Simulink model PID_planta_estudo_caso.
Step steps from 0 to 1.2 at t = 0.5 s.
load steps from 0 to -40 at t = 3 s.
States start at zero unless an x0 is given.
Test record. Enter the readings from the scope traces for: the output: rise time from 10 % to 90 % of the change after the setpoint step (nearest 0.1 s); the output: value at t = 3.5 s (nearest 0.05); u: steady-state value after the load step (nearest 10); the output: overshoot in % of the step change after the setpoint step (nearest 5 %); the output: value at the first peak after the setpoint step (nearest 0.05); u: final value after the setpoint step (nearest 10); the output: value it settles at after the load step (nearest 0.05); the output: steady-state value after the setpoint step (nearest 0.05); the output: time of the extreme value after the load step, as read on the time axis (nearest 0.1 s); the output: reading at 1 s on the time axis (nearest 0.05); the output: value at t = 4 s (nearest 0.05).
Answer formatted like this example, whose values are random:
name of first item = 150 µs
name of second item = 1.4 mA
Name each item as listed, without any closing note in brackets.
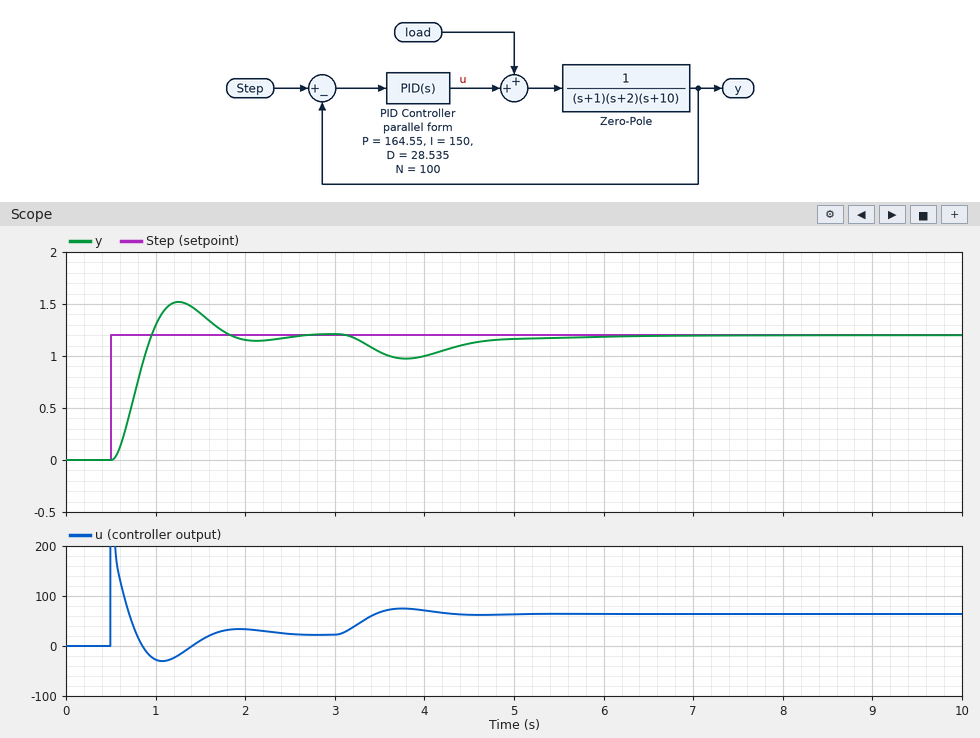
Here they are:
the output: rise time from 10 % to 90 % of the change after the setpoint step = 0.3 s
the output: value at t = 3.5 s = 1.05
u: steady-state value after the load step = 60
the output: overshoot in % of the step change after the setpoint step = 25 %
the output: value at the first peak after the setpoint step = 1.50
u: final value after the setpoint step = 20
the output: value it settles at after the load step = 1.20
the output: steady-state value after the setpoint step = 1.20
the output: time of the extreme value after the load step, as read on the time axis = 3.8 s
the output: reading at 1 s on the time axis = 1.30
the output: value at t = 4 s = 1.00
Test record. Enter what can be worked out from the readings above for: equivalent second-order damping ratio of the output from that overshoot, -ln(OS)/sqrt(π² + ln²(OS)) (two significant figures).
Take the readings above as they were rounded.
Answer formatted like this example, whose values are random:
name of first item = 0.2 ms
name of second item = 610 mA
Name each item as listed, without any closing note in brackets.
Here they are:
equivalent second-order damping ratio of the output from that overshoot, -ln(OS)/sqrt(π² + ln²(OS)) = 0.40
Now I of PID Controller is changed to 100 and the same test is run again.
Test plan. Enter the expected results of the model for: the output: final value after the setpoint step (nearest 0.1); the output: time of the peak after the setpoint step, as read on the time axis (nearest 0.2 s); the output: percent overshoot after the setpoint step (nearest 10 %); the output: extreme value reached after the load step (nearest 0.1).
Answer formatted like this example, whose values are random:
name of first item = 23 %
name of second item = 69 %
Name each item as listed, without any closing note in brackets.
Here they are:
the output: final value after the setpoint step = 1.2
the output: time of the peak after the setpoint step, as read on the time axis = 1.2 s
the output: percent overshoot after the setpoint step = 20 %
the output: extreme value reached after the load step = 1.0
